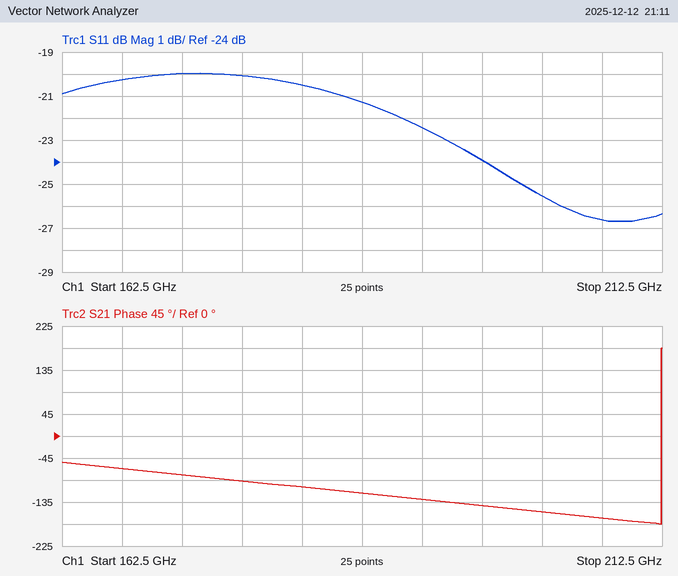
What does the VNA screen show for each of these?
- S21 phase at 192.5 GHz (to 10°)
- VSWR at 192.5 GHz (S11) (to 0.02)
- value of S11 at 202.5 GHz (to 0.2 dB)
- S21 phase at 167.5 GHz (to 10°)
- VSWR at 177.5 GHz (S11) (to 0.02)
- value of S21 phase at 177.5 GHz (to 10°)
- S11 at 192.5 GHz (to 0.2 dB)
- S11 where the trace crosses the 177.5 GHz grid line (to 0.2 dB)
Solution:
-130°
1.16
-25.6 dB
-70°
1.22
-90°
-22.4 dB
-20.0 dB
